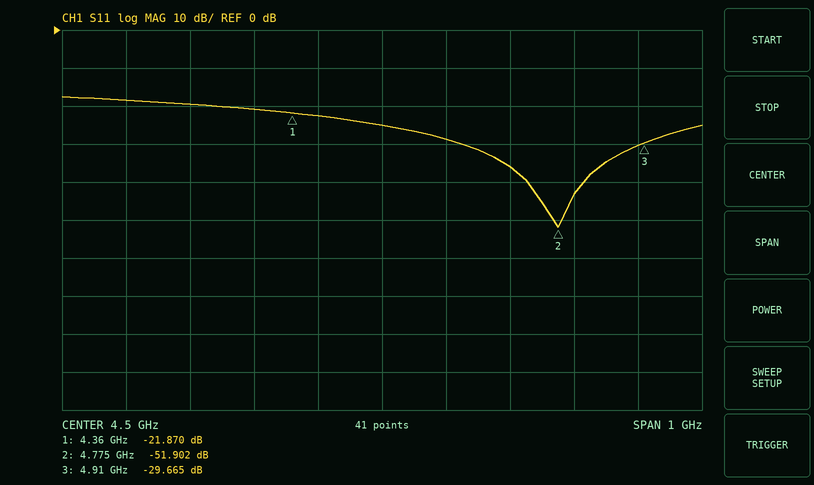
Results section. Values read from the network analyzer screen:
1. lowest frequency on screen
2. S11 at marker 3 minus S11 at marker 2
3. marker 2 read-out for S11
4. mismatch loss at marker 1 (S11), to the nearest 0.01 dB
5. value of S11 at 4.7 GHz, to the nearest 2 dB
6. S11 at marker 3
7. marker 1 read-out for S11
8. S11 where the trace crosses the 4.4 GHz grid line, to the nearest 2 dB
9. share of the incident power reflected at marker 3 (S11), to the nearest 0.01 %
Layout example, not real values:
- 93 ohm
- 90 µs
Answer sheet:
- 4 GHz
- 22.237 dB
- -51.902 dB
- 0.03 dB
- -36 dB
- -29.665 dB
- -21.870 dB
- -22 dB
- 0.11 %
